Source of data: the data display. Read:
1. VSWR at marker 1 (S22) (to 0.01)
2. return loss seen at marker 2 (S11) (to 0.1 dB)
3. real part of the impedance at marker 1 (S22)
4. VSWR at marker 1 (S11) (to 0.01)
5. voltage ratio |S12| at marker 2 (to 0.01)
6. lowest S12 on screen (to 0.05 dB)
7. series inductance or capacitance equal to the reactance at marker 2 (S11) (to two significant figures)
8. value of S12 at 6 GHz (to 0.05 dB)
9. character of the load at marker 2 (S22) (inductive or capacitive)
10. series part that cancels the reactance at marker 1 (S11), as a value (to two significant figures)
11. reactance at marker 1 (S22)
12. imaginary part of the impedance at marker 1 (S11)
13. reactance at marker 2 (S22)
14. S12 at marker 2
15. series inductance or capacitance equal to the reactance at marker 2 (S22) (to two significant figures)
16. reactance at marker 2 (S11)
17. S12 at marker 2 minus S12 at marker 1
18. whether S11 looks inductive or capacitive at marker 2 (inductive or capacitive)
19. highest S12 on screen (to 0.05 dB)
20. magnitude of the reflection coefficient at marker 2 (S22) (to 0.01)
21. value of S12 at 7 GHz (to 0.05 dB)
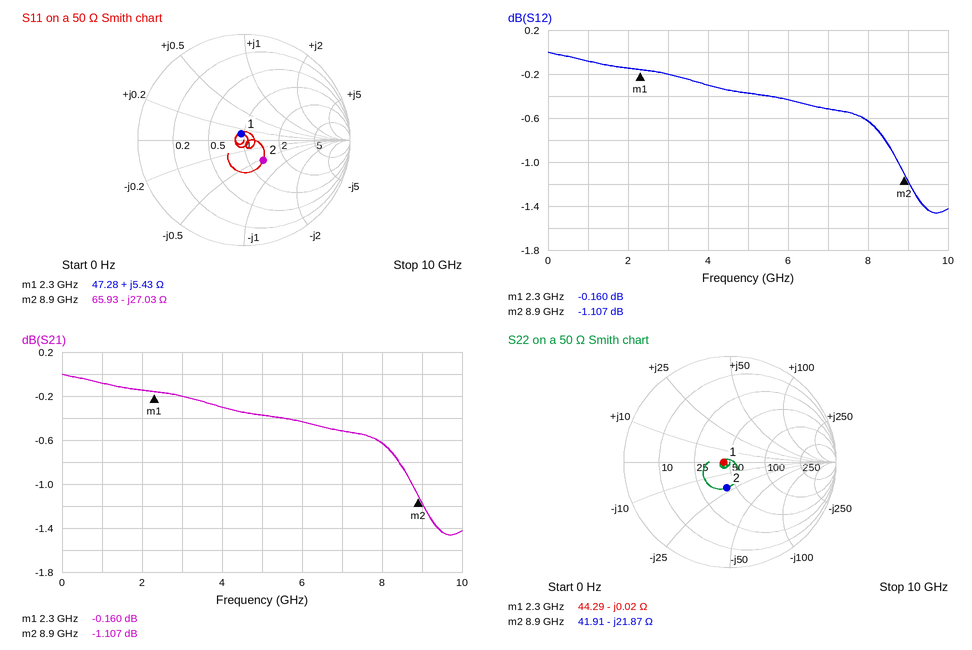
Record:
1.13
11.6 dB
44.29 Ω
1.13
0.88
-1.45 dB
660 fF
-0.45 dB
capacitive
13 pF
-0.02 Ω
+5.43 Ω
-21.87 Ω
-1.107 dB
820 fF
-27.03 Ω
-0.947 dB
capacitive
0.00 dB
0.25
-0.50 dB
